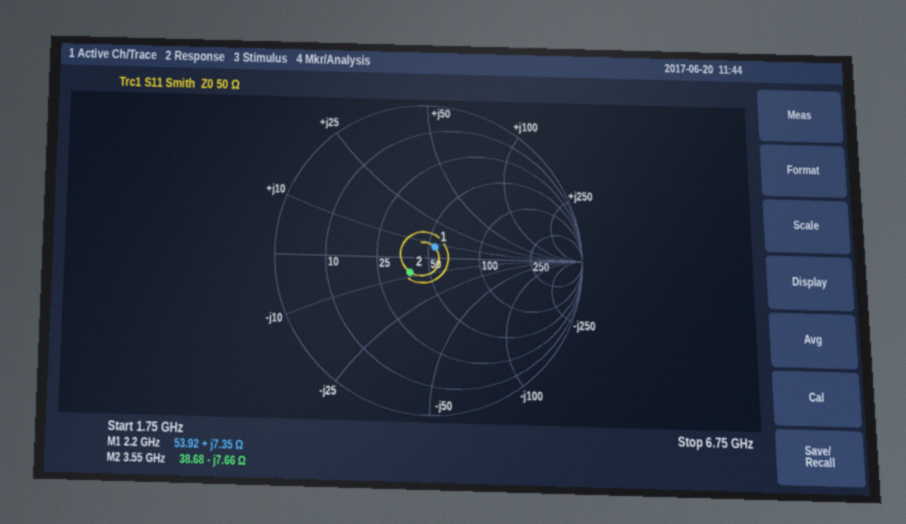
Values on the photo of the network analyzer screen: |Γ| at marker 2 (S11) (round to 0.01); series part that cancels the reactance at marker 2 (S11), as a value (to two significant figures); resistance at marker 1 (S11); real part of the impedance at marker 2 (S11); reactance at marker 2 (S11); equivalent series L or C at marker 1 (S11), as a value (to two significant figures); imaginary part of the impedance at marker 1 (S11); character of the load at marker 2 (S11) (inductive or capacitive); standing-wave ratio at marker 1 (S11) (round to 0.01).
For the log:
0.15
340 pH
53.92 Ω
38.68 Ω
-7.66 Ω
530 pH
+7.35 Ω
capacitive
1.17
